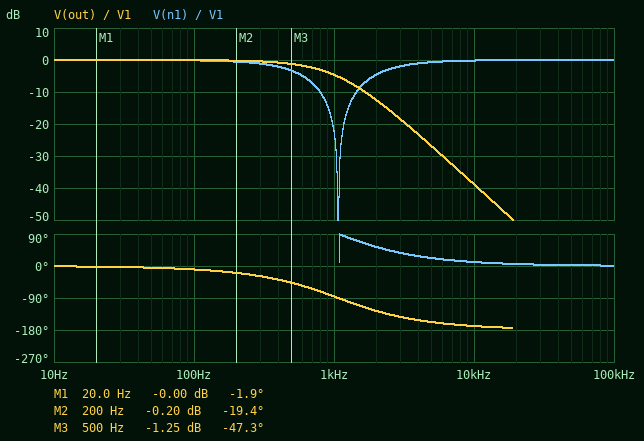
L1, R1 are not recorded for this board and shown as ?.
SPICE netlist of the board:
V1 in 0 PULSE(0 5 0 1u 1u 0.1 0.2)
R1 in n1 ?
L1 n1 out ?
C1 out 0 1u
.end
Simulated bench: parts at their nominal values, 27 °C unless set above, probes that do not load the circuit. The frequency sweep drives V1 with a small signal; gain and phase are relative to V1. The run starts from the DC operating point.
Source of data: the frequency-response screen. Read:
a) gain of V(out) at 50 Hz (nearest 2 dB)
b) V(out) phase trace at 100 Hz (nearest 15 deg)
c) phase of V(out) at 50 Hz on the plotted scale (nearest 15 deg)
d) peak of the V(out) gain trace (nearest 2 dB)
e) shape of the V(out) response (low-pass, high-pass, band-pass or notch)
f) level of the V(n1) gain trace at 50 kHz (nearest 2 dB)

0 dB
-15 deg
0 deg
0 dB
low-pass
0 dB
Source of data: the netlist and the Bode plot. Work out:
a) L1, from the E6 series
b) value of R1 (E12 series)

22 mH
270 Ω
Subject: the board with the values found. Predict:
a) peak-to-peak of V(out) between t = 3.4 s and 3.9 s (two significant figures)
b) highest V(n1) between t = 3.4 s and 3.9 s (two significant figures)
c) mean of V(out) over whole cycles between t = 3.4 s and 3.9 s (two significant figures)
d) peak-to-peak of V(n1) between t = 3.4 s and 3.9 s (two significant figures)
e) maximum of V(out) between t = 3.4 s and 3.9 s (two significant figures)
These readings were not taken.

5.0 V
5.0 V
2.5 V
5.0 V
5.0 V
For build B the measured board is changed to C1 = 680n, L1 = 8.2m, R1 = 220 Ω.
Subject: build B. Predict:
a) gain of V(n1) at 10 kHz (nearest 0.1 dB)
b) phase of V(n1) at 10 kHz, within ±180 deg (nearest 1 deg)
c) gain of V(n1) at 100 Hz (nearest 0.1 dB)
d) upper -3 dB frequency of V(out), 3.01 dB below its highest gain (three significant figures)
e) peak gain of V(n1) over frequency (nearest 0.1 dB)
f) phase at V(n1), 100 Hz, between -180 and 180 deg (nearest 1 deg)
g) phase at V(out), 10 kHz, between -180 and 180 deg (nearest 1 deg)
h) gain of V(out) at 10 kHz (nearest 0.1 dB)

-0.8 dB
24 deg
0 dB
1.37 kHz
0 dB
-5 deg
-156 deg
-27.2 dB
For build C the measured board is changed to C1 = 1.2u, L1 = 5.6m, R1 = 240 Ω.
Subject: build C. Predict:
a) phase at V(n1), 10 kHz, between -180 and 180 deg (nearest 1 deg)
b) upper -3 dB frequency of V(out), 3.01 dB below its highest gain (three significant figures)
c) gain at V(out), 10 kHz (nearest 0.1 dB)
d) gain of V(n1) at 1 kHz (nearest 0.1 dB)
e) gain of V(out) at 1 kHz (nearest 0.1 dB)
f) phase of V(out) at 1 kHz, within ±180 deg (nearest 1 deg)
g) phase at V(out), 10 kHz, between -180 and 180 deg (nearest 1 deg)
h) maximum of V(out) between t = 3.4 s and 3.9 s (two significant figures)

35 deg
601 Hz
-29.9 dB
-8.5 dB
-5.8 dB
-68 deg
-145 deg
5.0 V
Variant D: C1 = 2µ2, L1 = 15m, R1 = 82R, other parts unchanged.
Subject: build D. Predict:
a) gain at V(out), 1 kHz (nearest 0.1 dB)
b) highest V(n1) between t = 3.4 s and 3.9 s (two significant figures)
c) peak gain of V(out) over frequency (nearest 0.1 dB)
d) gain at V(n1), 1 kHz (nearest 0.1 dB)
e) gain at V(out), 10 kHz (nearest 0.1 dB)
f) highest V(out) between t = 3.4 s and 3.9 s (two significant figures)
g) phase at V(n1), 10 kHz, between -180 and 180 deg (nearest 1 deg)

-1.4 dB
5.5 V
1.3 dB
-11.8 dB
-42.3 dB
5.9 V
5 deg
